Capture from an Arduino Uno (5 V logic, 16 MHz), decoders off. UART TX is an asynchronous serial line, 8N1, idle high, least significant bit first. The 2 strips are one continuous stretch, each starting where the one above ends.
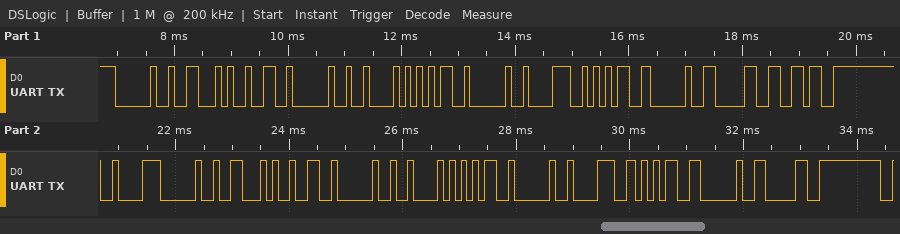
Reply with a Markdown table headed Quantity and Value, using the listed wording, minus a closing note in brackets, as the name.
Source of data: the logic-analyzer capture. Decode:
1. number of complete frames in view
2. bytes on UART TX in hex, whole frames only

| Quantity | Value |
|---|---|
| number of complete frames in view | 24 |
| bytes on UART TX in hex, whole frames only | 0x20 0x46 0x32 0x20 0x42 0x35 0x20 0x38 0x35 0x20 0x30 0x36 0xC2 0x20 0x46 0x32 0x20 0x42 0x35 0x20 0x38 0x35 0x20 0x30 |
